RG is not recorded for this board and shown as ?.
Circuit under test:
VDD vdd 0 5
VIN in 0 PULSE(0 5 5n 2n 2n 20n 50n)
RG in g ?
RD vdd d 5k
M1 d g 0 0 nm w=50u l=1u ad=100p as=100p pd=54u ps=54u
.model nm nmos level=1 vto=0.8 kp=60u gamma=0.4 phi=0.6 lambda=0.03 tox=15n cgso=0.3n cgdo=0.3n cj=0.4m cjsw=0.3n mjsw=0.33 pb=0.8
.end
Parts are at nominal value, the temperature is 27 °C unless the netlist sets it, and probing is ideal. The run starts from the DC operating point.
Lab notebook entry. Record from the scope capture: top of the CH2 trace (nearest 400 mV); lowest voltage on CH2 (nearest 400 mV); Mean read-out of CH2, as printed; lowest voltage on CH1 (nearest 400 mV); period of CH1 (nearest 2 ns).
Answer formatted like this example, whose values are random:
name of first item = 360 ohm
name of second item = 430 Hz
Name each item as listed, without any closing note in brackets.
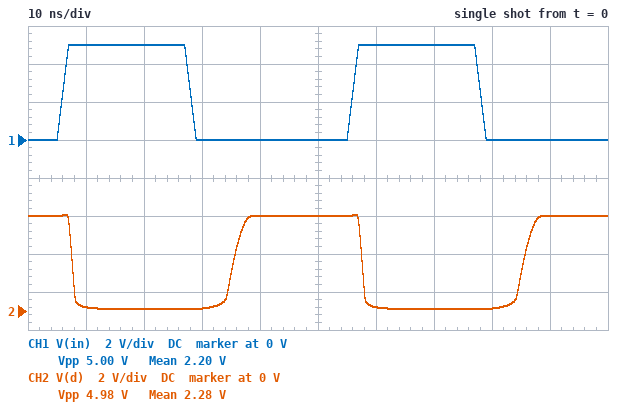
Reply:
top of the CH2 trace = 5.2 V
lowest voltage on CH2 = 0 V
Mean read-out of CH2, as printed = 2.28 V
lowest voltage on CH1 = 0 V
period of CH1 = 50 ns
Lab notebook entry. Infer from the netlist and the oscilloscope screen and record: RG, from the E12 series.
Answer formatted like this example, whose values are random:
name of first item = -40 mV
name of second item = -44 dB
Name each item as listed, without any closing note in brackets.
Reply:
RG, from the E12 series = 33 kΩ
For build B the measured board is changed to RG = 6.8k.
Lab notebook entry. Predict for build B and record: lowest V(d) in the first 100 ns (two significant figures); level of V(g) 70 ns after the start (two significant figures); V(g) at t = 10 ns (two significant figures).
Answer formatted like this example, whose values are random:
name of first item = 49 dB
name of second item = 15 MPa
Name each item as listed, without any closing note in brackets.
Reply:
lowest V(d) in the first 100 ns = 77 mV
level of V(g) 70 ns after the start = 5.0 V
V(g) at t = 10 ns = 4.9 V
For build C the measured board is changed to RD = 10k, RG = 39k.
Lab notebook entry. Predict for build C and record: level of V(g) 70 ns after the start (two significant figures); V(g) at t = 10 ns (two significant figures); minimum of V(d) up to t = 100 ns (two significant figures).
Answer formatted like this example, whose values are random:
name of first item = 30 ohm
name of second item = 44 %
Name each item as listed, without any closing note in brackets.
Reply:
level of V(g) 70 ns after the start = 4.5 V
V(g) at t = 10 ns = 2.3 V
minimum of V(d) up to t = 100 ns = 40 mV
